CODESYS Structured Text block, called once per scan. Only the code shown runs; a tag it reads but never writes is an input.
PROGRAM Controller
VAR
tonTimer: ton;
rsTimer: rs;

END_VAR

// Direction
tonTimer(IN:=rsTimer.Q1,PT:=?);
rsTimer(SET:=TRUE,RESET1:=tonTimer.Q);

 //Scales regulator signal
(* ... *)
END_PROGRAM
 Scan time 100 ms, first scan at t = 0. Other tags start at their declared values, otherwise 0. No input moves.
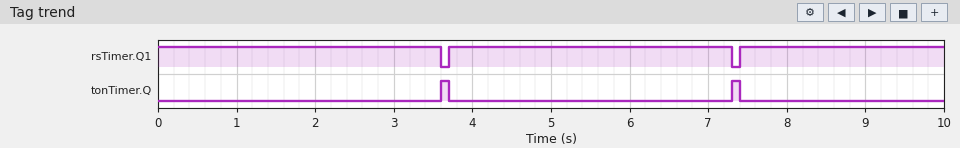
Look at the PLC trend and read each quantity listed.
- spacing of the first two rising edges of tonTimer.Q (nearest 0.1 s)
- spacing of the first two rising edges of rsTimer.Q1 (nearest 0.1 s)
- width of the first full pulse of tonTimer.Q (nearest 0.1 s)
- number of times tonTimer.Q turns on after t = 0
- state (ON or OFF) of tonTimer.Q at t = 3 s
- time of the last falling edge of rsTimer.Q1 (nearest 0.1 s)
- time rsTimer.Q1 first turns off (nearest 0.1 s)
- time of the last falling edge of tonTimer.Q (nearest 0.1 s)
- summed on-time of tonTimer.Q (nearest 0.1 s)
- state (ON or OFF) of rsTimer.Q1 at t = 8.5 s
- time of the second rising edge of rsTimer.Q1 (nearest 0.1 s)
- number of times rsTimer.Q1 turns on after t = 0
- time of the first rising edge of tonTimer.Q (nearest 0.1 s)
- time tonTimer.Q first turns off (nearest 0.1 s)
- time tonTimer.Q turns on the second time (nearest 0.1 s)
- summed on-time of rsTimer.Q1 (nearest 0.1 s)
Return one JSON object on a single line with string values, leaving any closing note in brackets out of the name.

{"spacing of the first two rising edges of tonTimer.Q": "3.7 s", "spacing of the first two rising edges of rsTimer.Q1": "3.7 s", "width of the first full pulse of tonTimer.Q": "0.1 s", "number of times tonTimer.Q turns on after t = 0": "2", "state (ON or OFF) of tonTimer.Q at t = 3 s": "OFF", "time of the last falling edge of rsTimer.Q1": "7.3 s", "time rsTimer.Q1 first turns off": "3.6 s", "time of the last falling edge of tonTimer.Q": "7.4 s", "summed on-time of tonTimer.Q": "0.2 s", "state (ON or OFF) of rsTimer.Q1 at t = 8.5 s": "ON", "time of the second rising edge of rsTimer.Q1": "7.4 s", "number of times rsTimer.Q1 turns on after t = 0": "2", "time of the first rising edge of tonTimer.Q": "3.6 s", "time tonTimer.Q first turns off": "3.7 s", "time tonTimer.Q turns on the second time": "7.3 s", "summed on-time of rsTimer.Q1": "9.8 s"}
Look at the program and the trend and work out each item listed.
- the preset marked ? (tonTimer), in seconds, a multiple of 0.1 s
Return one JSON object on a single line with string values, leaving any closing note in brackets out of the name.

{"the preset marked ? (tonTimer), in seconds, a multiple of 0.1 s": "3.5 s"}
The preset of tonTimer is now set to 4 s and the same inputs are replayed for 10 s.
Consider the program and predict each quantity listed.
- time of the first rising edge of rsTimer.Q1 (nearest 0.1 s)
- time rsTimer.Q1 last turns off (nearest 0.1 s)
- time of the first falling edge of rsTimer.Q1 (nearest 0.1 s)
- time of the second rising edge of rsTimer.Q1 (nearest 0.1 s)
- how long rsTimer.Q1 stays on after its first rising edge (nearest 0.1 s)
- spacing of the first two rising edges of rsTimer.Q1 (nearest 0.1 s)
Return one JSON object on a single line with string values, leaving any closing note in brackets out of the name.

{"time of the first rising edge of rsTimer.Q1": "4.2 s", "time rsTimer.Q1 last turns off": "8.3 s", "time of the first falling edge of rsTimer.Q1": "4.1 s", "time of the second rising edge of rsTimer.Q1": "8.4 s", "how long rsTimer.Q1 stays on after its first rising edge": "4.1 s", "spacing of the first two rising edges of rsTimer.Q1": "4.2 s"}
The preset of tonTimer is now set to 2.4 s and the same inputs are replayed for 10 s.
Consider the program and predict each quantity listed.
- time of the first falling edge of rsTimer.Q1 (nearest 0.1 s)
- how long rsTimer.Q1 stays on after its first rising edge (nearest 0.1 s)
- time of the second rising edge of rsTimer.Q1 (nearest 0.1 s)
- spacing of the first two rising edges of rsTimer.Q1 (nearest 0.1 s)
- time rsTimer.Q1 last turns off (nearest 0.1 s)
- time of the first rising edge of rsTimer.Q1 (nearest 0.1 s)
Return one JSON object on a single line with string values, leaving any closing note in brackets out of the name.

{"time of the first falling edge of rsTimer.Q1": "2.5 s", "how long rsTimer.Q1 stays on after its first rising edge": "2.5 s", "time of the second rising edge of rsTimer.Q1": "5.2 s", "spacing of the first two rising edges of rsTimer.Q1": "2.6 s", "time rsTimer.Q1 last turns off": "7.7 s", "time of the first rising edge of rsTimer.Q1": "2.6 s"}
